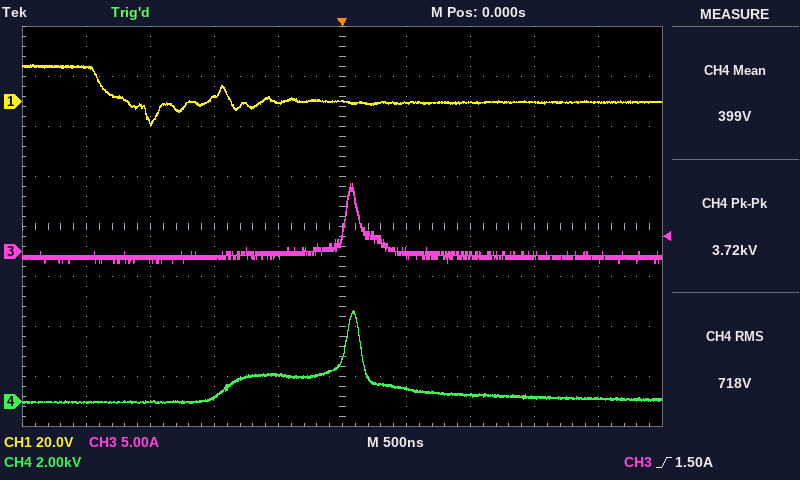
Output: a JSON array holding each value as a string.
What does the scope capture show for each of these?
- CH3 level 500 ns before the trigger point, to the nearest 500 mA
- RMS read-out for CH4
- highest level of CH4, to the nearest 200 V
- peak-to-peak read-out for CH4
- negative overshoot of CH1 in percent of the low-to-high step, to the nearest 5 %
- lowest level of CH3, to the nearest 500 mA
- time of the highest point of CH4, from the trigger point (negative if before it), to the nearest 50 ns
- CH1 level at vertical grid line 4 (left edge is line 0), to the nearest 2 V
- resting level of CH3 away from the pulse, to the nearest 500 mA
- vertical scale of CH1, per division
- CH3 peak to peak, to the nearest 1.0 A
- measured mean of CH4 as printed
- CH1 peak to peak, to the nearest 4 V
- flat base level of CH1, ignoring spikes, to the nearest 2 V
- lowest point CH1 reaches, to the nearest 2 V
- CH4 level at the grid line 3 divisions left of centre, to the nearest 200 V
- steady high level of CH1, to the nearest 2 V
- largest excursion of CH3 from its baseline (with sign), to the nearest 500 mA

["-500 mA", "718 V", "3.6 kV", "3.72 kV", "65 %", "-1.0 A", "+100 ns", "0 V", "-500 mA", "20 V", "8.0 A", "399 V", "24 V", "0 V", "-10 V", "0.0 kV", "14 V", "+7.5 A"]
